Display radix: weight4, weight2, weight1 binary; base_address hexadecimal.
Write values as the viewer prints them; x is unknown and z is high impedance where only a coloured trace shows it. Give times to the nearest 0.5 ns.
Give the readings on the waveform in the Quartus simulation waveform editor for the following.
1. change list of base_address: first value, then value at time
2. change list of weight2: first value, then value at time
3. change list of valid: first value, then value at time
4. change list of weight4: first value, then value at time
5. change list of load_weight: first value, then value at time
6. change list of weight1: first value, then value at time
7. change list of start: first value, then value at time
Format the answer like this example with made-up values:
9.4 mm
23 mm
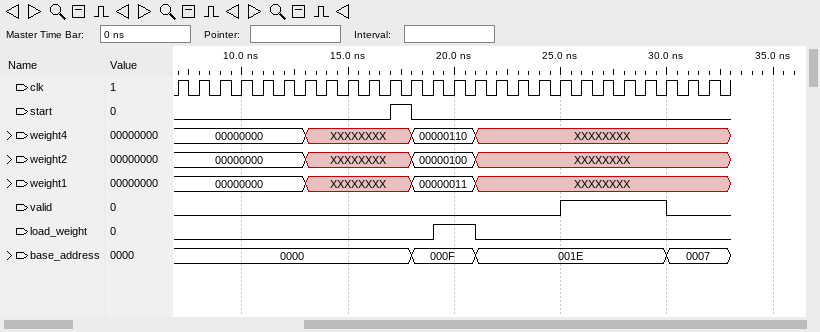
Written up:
0000, 000F at 18 ns, 001E at 21 ns, 0007 at 30 ns
00000000, XXXXXXXX at 13 ns, 00000100 at 18 ns, XXXXXXXX at 21 ns
0, 1 at 25 ns, 0 at 30 ns
00000000, XXXXXXXX at 13 ns, 00000110 at 18 ns, XXXXXXXX at 21 ns
0, 1 at 19 ns, 0 at 21 ns
00000000, XXXXXXXX at 13 ns, 00000011 at 18 ns, XXXXXXXX at 21 ns
0, 1 at 17 ns, 0 at 18 ns
